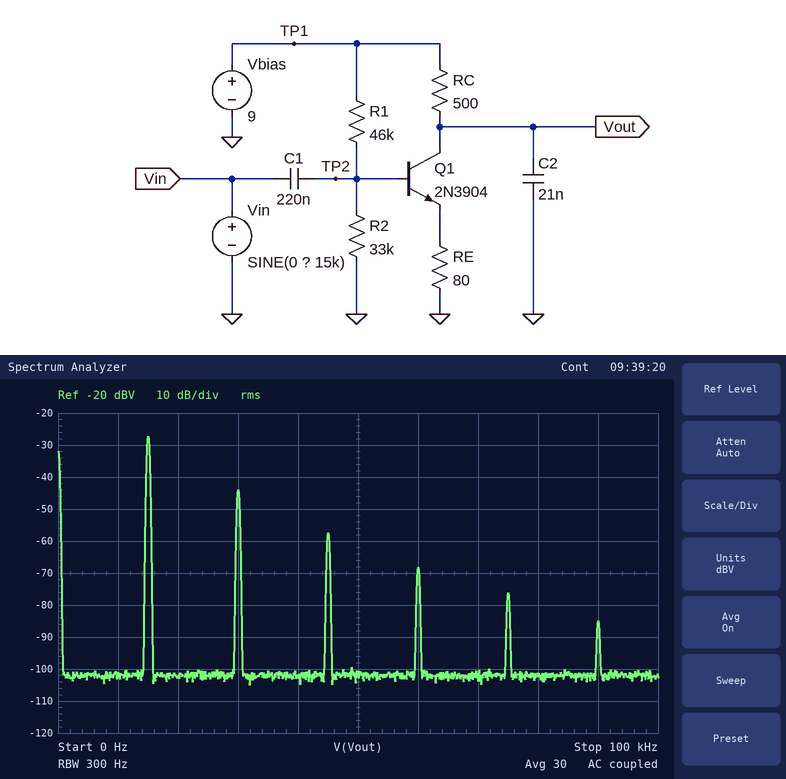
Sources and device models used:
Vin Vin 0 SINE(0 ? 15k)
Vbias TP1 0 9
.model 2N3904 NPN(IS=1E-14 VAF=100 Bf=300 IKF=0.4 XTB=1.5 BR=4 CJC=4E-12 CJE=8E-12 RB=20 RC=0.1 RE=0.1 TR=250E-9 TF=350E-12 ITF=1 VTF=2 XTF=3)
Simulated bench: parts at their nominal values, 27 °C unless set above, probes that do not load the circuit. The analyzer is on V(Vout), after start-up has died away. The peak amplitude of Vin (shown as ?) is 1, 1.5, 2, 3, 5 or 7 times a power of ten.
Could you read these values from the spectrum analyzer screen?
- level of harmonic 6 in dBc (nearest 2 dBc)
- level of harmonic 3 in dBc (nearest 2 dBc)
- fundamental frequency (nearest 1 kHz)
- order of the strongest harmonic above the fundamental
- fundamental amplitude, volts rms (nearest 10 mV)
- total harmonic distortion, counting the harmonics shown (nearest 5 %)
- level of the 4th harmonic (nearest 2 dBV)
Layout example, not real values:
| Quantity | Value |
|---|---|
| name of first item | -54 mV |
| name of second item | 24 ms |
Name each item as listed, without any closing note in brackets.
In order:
| Quantity | Value |
|---|---|
| level of harmonic 6 in dBc | -58 dBc |
| level of harmonic 3 in dBc | -30 dBc |
| fundamental frequency | 15 kHz |
| order of the strongest harmonic above the fundamental | 2 |
| fundamental amplitude, volts rms | 40 mV |
| total harmonic distortion, counting the harmonics shown | 15 % |
| level of the 4th harmonic | -68 dBV |
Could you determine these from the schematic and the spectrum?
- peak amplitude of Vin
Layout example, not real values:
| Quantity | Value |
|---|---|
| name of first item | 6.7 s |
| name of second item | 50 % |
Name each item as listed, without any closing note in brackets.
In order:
| Quantity | Value |
|---|---|
| peak amplitude of Vin | 20 mV |
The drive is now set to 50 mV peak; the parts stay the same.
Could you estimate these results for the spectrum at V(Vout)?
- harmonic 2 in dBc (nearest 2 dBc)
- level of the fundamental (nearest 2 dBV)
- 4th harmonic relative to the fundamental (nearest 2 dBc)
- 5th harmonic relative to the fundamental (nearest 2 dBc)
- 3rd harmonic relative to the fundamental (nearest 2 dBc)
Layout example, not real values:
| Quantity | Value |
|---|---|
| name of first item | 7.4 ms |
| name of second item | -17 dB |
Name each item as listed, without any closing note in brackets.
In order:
| Quantity | Value |
|---|---|
| harmonic 2 in dBc | -20 dBc |
| level of the fundamental | -18 dBV |
| 4th harmonic relative to the fundamental | -36 dBc |
| 5th harmonic relative to the fundamental | -44 dBc |
| 3rd harmonic relative to the fundamental | -28 dBc |
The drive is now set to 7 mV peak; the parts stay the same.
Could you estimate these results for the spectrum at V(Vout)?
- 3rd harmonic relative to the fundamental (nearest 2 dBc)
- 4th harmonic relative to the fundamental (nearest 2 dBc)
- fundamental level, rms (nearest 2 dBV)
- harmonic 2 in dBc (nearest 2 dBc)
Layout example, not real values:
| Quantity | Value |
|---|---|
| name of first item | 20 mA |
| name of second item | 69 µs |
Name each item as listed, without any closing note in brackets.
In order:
| Quantity | Value |
|---|---|
| 3rd harmonic relative to the fundamental | -42 dBc |
| 4th harmonic relative to the fundamental | -58 dBc |
| fundamental level, rms | -38 dBV |
| harmonic 2 in dBc | -20 dBc |
